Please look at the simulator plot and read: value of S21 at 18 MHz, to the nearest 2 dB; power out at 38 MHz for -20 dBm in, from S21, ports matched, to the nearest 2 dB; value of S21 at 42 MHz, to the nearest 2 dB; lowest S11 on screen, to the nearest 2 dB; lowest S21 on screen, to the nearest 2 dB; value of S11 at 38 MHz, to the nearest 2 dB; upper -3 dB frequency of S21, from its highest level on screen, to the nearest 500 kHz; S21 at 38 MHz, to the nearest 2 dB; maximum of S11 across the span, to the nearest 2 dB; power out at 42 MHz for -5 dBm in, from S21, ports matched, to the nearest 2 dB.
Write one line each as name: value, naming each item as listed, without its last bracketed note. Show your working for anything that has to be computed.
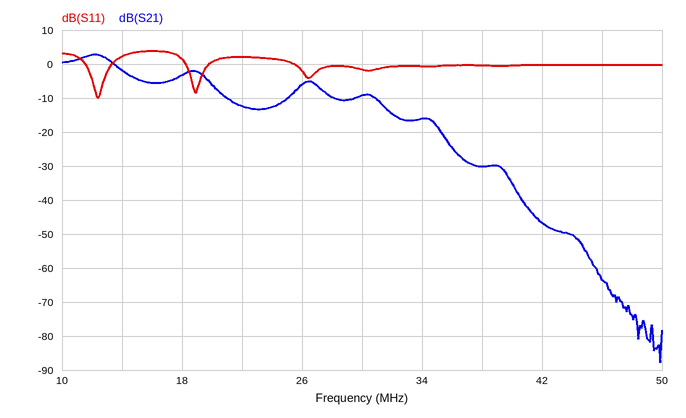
value of S21 at 18 MHz, to the nearest 2 dB: -4 dB
power out at 38 MHz for -20 dBm in, from S21, ports matched, to the nearest 2 dB: -20 dBm + (-30 dB) = -50 dBm
value of S21 at 42 MHz, to the nearest 2 dB: -46 dB
lowest S11 on screen, to the nearest 2 dB: -10 dB
lowest S21 on screen, to the nearest 2 dB: -88 dB
value of S11 at 38 MHz, to the nearest 2 dB: 0 dB
upper -3 dB frequency of S21, from its highest level on screen, to the nearest 500 kHz: 13.5 MHz
S21 at 38 MHz, to the nearest 2 dB: -30 dB
maximum of S11 across the span, to the nearest 2 dB: 4 dB
power out at 42 MHz for -5 dBm in, from S21, ports matched, to the nearest 2 dB: -5 dBm + (-46 dB) = -52 dBm
